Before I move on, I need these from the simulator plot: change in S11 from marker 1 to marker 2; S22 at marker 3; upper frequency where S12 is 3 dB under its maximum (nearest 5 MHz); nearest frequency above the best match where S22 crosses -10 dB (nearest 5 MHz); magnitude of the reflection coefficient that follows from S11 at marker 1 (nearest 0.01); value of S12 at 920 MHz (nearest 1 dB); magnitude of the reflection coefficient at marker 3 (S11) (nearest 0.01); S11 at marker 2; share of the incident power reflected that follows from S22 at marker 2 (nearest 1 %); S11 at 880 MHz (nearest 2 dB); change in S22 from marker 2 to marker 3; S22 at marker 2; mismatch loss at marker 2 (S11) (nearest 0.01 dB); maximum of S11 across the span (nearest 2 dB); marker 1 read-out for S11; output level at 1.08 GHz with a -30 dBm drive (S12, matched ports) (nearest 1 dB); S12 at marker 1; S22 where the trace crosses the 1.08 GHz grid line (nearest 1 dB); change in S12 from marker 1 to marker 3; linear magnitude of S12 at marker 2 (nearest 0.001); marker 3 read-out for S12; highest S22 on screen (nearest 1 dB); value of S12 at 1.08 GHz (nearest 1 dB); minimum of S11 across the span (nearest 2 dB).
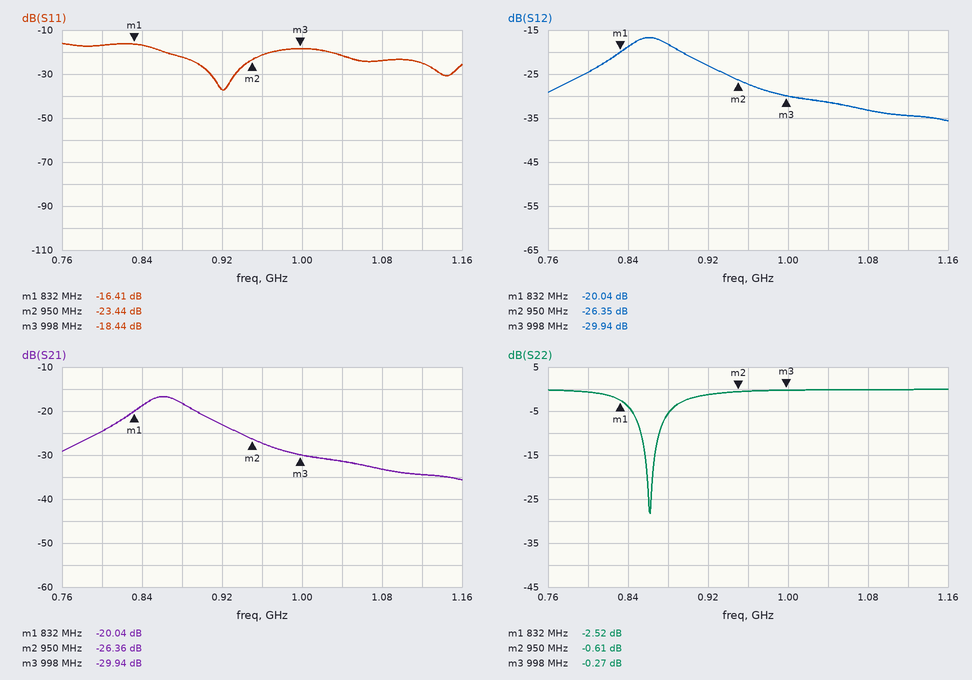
-7.03 dB
-0.27 dB
890 MHz
870 MHz
0.15
-23 dB
0.12
-23.44 dB
87 %
-22 dB
0.34 dB
-0.61 dB
0.02 dB
-16 dB
-16.41 dB
-63 dBm
-20.04 dB
0 dB
-9.90 dB
0.048
-29.94 dB
0 dB
-33 dB
-38 dB
